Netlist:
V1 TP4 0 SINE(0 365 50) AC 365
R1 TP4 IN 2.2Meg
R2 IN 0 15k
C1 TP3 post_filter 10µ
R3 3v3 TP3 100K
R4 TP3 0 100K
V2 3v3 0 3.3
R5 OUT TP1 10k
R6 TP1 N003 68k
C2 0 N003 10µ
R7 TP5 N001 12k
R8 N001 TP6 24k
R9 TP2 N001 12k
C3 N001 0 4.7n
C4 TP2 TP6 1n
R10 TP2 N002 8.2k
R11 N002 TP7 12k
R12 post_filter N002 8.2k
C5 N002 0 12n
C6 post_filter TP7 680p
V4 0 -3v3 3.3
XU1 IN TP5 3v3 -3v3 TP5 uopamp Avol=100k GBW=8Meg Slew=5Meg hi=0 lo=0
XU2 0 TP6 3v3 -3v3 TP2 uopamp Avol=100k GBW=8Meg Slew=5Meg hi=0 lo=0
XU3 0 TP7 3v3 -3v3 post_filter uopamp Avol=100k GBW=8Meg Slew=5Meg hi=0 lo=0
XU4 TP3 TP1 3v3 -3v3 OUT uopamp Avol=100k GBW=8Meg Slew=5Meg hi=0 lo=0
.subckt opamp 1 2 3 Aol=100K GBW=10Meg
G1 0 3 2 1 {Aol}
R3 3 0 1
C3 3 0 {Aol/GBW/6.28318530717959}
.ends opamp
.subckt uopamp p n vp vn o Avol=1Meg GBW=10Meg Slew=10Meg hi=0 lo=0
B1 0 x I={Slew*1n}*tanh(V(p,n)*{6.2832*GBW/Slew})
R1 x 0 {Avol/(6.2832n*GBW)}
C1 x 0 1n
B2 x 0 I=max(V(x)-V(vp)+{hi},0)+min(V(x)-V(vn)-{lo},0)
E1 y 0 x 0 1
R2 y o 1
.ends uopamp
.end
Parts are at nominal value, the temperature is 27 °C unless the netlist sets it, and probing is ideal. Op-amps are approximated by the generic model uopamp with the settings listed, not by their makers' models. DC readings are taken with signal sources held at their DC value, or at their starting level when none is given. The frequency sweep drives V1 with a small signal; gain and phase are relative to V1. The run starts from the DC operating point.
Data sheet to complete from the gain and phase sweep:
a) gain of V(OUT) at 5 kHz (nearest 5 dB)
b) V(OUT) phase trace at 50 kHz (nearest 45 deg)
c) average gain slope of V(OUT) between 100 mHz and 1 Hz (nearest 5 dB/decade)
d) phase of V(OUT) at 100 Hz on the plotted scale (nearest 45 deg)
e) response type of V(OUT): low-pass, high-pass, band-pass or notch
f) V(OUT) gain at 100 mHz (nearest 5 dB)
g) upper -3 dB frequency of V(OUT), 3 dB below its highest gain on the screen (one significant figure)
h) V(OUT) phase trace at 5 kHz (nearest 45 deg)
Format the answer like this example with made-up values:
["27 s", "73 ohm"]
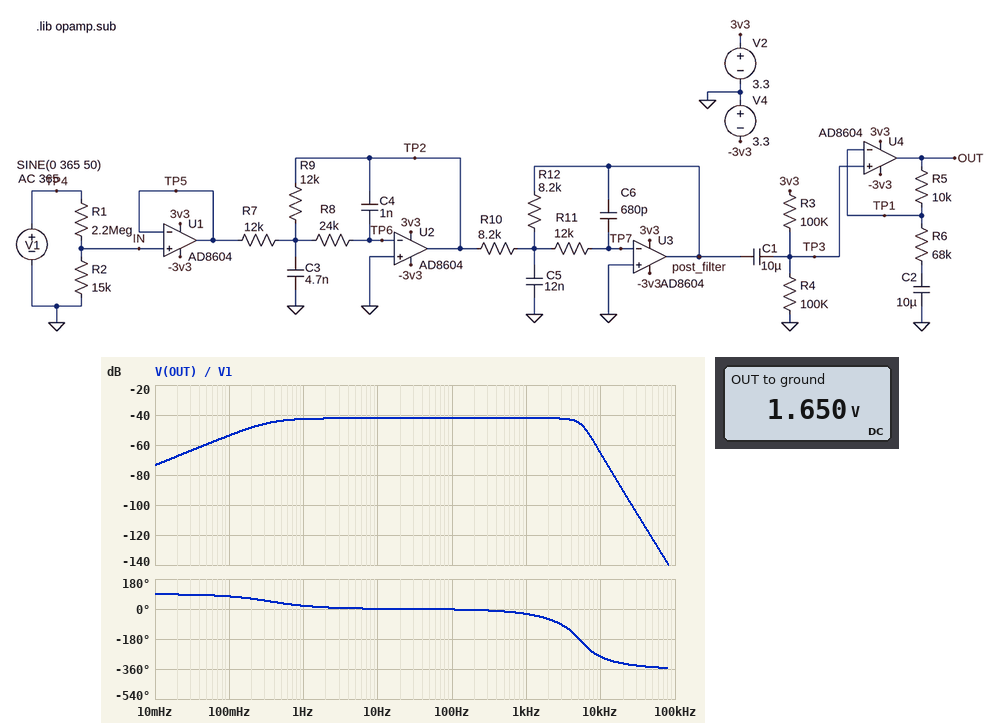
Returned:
["-45 dB", "-360 deg", "10 dB/decade", "0 deg", "band-pass", "-55 dB", "5 kHz", "-180 deg"]
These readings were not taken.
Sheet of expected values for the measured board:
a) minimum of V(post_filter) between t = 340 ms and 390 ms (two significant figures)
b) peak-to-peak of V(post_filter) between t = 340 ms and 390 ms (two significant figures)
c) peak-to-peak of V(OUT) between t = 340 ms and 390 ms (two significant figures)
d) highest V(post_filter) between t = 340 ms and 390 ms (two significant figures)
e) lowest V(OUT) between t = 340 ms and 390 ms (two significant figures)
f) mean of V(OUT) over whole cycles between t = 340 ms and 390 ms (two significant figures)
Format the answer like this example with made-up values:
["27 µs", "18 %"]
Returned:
["-2.5 V", "4.9 V", "4.5 V", "2.5 V", "-1.2 V", "1.4 V"]
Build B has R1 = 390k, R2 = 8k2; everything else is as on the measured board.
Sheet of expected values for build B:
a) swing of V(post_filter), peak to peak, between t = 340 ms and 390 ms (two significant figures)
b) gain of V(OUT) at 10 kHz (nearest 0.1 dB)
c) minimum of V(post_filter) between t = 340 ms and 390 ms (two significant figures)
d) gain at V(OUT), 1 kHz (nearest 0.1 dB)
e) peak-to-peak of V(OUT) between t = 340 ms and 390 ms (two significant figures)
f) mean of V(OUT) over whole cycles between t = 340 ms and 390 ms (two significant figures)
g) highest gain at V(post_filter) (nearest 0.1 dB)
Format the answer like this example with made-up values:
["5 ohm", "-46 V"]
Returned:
["6.6 V", "-56.0 dB", "-3.3 V", "-32.5 dB", "5.4 V", "820 mV", "-33.7 dB"]
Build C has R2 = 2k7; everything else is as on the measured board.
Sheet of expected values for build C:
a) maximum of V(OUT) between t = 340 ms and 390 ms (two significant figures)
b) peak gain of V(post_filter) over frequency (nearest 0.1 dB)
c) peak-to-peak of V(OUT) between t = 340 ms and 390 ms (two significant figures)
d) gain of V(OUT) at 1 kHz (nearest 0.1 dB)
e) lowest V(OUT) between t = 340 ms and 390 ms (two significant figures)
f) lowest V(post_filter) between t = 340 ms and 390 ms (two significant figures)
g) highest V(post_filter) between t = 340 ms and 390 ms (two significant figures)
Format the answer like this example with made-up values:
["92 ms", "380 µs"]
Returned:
["2.2 V", "-58.2 dB", "1.0 V", "-57.0 dB", "1.1 V", "-450 mV", "450 mV"]
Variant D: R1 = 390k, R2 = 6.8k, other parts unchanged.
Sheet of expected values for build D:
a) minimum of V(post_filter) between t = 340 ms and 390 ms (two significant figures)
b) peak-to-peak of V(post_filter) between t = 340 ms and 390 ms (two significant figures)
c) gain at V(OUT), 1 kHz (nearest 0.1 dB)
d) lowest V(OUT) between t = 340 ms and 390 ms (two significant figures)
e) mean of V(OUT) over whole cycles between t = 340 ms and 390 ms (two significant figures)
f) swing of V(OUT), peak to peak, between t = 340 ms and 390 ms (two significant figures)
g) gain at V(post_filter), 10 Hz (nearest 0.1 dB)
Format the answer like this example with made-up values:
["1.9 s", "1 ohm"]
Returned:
["-3.3 V", "6.6 V", "-34.1 dB", "-2.1 V", "870 mV", "5.4 V", "-35.3 dB"]
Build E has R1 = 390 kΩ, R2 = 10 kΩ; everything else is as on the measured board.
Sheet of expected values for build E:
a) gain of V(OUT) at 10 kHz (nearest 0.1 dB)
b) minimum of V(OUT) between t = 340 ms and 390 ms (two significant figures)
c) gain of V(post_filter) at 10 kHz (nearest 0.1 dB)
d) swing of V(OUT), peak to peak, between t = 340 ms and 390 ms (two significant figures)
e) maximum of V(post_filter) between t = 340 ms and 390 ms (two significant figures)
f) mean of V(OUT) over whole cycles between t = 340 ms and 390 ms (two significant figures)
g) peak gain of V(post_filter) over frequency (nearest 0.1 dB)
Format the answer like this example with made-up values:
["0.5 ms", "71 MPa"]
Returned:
["-54.3 dB", "-2.1 V", "-55.5 dB", "5.4 V", "3.3 V", "780 mV", "-32.0 dB"]
